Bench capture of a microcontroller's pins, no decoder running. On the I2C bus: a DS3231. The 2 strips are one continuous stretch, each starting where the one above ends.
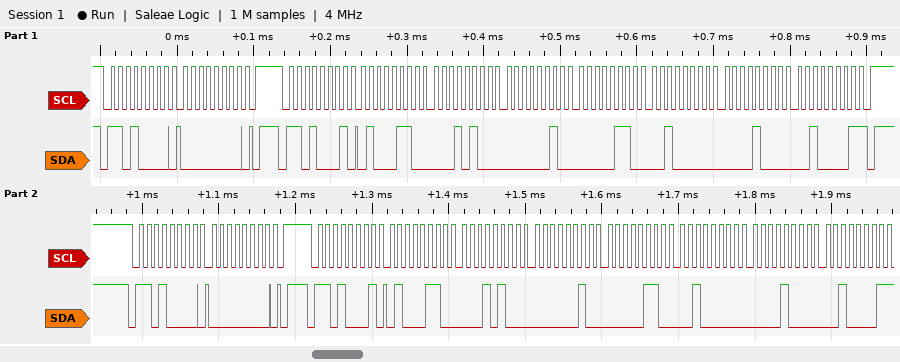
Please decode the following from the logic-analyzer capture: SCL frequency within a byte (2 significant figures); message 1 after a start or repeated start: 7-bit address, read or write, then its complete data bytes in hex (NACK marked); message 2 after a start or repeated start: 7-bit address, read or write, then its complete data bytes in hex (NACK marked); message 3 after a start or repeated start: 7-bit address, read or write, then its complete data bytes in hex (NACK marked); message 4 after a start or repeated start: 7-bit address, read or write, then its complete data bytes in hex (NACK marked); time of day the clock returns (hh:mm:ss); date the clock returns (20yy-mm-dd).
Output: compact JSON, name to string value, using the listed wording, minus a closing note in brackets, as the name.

{"SCL frequency within a byte": "100 kHz", "message 1 after a start or repeated start: 7-bit address, read or write, then its complete data bytes in hex": "0x68 write: 00", "message 2 after a start or repeated start: 7-bit address, read or write, then its complete data bytes in hex": "0x68 read: 46 14 02 06 20 08 21 NACK", "message 3 after a start or repeated start: 7-bit address, read or write, then its complete data bytes in hex": "0x68 write: 00", "message 4 after a start or repeated start: 7-bit address, read or write, then its complete data bytes in hex": "0x68 read: 46 14 02 06 20 08 21 NACK", "time of day the clock returns": "02:14:46", "date the clock returns": "2021-08-20"}
